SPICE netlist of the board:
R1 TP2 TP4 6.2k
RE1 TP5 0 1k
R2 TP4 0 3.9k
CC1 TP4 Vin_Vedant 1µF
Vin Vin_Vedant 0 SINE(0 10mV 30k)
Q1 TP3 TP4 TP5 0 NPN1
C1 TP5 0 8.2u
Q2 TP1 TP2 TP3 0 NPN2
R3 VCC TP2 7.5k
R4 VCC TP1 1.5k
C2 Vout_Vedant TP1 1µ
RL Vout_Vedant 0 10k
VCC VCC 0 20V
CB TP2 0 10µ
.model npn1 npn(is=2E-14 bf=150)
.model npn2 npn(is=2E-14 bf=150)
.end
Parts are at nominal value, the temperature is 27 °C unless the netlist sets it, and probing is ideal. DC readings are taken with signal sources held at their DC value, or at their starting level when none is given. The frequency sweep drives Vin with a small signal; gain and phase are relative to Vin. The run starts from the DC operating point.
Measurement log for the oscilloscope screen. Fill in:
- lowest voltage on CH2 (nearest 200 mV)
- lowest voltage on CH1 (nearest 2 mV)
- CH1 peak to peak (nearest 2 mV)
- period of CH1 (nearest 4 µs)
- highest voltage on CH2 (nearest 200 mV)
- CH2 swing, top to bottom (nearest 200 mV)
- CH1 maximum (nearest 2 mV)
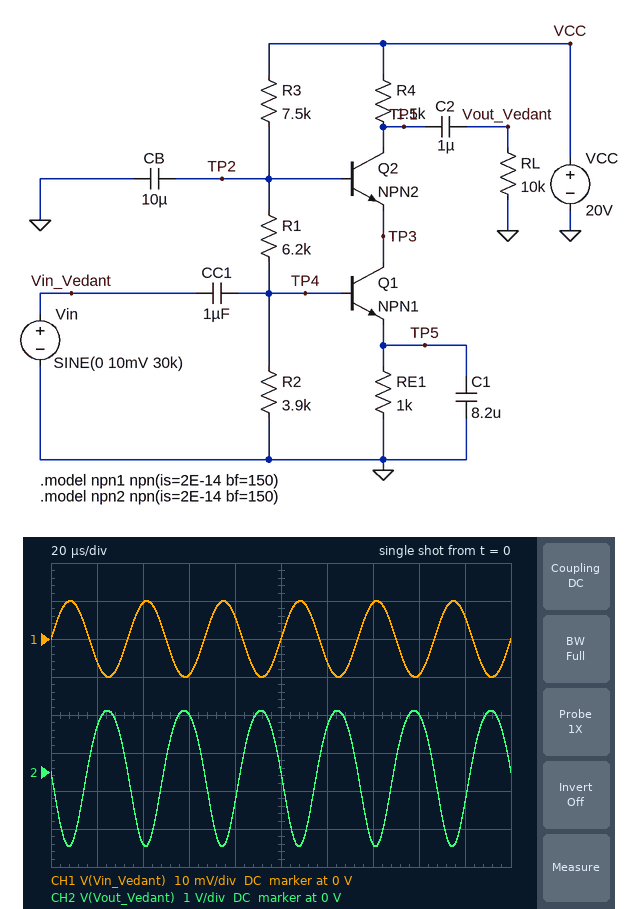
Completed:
-2.0 V
-10 mV
20 mV
32 µs
1.6 V
3.6 V
10 mV
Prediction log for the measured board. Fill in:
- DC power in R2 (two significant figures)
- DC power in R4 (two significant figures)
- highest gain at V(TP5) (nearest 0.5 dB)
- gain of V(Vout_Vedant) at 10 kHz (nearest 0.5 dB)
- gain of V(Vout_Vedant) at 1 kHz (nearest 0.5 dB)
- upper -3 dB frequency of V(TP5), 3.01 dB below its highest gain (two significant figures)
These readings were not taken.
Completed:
4.8 mW
19 mW
-0.5 dB
45.0 dB
35.5 dB
3.0 kHz
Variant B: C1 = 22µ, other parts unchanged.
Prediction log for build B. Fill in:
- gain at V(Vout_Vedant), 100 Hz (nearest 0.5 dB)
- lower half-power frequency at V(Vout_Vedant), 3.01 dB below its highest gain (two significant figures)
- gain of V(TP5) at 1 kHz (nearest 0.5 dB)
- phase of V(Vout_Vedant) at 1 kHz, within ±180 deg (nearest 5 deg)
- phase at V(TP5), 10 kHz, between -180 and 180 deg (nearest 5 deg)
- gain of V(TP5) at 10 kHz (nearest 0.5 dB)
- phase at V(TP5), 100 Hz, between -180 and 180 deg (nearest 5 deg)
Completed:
22.5 dB
1.2 kHz
-3.5 dB
-125 deg
-85 deg
-20.0 dB
25 deg
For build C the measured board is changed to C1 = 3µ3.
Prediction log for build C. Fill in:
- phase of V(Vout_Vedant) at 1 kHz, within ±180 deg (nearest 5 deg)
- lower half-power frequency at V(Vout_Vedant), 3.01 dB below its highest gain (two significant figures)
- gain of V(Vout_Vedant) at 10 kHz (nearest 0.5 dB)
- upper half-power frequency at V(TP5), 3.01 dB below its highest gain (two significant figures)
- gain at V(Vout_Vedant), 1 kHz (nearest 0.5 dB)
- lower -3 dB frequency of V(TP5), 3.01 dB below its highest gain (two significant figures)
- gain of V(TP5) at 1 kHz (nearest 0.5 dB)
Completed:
-95 deg
7.0 kHz
43.5 dB
7.1 kHz
28.0 dB
66 Hz
-0.5 dB
